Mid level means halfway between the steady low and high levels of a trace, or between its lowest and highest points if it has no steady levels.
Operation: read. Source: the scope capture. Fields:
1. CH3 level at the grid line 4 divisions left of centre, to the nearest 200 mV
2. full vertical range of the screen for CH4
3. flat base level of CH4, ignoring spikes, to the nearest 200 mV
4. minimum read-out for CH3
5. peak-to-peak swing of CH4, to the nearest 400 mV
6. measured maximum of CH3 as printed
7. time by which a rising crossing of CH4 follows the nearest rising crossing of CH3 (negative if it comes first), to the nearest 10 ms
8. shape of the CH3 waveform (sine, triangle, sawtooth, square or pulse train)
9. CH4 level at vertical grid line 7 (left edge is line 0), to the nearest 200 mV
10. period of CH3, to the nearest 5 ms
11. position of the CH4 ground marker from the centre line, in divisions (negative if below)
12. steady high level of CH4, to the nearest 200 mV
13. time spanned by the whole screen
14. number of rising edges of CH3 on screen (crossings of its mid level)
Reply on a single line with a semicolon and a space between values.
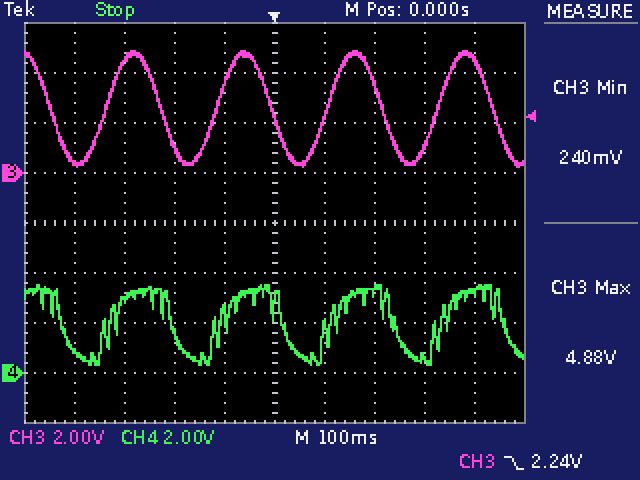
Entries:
400 mV; 16 V; 600 mV; 240 mV; 3.2 V; 4.88 V; +10 ms; sine; 3.2 V; 220 ms; -3.0 div; 3.2 V; 1 s; 4
